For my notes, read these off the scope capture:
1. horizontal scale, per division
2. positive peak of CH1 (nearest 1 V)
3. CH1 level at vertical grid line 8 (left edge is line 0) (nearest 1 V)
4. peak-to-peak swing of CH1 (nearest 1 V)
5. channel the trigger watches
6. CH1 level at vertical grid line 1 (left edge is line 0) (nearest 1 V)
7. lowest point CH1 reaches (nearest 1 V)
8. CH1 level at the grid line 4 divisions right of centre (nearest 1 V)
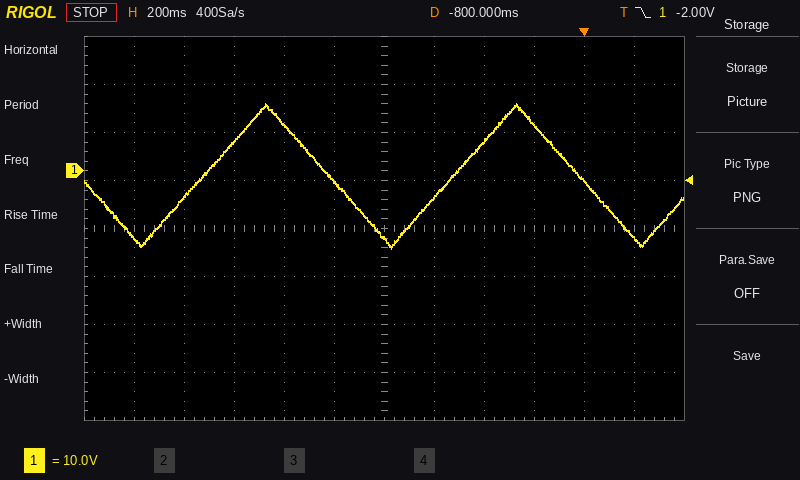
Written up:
200 ms
14 V
6 V
30 V
CH1
-14 V
-16 V
-2 V
